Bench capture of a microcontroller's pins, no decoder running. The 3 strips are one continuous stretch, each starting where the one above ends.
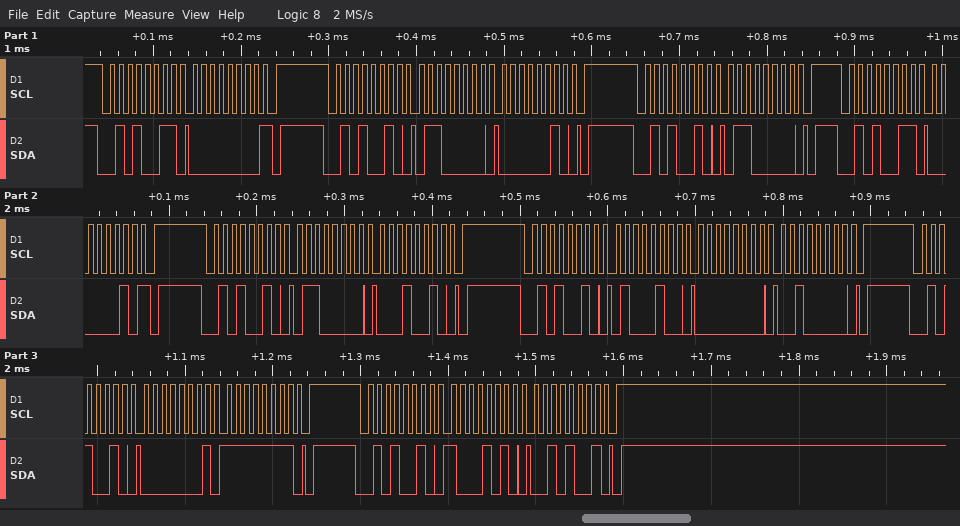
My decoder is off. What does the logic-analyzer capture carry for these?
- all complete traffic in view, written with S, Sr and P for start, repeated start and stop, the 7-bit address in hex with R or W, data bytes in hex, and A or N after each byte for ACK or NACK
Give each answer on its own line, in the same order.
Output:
S 29R A 00 N P S 29W A 60 A 02 A P S 29W A 60 A P S 29R A 02 N P S 29W A 60 A 12 A P S 29W A 44 A 00 A 20 A P S 29W A 01 A FF A P S 29W A 8A A 29 A P
